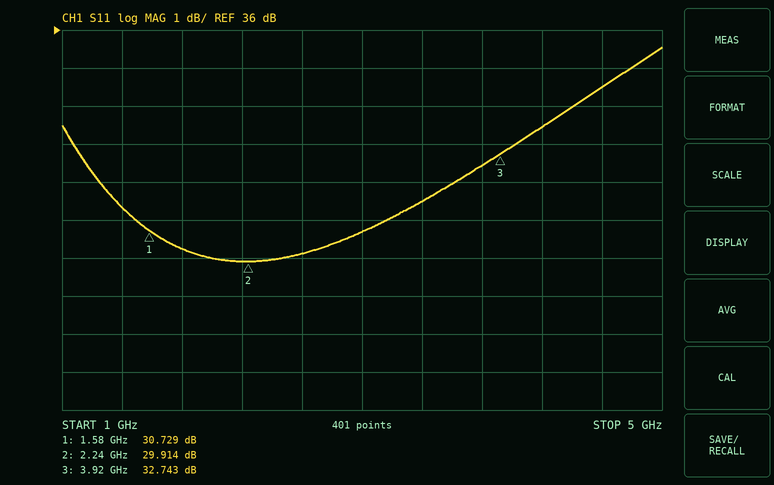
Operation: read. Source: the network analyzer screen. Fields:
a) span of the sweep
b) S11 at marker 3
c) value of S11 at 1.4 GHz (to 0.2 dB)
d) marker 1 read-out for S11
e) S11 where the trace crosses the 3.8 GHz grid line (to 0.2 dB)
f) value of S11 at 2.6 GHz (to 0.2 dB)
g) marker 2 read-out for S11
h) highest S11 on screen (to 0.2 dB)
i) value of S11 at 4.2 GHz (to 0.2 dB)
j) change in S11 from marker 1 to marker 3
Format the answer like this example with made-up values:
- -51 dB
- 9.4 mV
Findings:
- 4 GHz
- 32.743 dB
- 31.4 dB
- 30.729 dB
- 32.4 dB
- 30.2 dB
- 29.914 dB
- 35.6 dB
- 33.4 dB
- 2.014 dB
